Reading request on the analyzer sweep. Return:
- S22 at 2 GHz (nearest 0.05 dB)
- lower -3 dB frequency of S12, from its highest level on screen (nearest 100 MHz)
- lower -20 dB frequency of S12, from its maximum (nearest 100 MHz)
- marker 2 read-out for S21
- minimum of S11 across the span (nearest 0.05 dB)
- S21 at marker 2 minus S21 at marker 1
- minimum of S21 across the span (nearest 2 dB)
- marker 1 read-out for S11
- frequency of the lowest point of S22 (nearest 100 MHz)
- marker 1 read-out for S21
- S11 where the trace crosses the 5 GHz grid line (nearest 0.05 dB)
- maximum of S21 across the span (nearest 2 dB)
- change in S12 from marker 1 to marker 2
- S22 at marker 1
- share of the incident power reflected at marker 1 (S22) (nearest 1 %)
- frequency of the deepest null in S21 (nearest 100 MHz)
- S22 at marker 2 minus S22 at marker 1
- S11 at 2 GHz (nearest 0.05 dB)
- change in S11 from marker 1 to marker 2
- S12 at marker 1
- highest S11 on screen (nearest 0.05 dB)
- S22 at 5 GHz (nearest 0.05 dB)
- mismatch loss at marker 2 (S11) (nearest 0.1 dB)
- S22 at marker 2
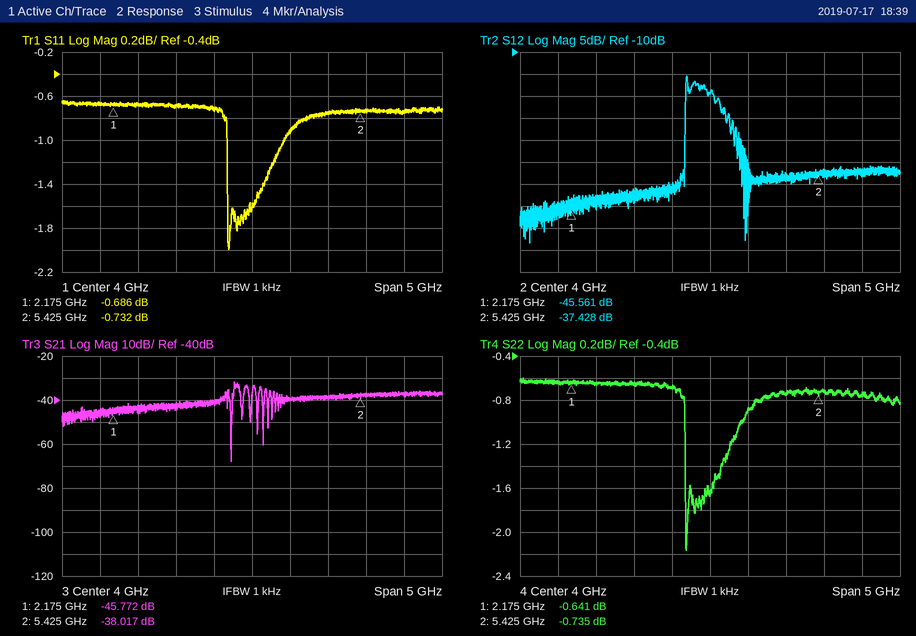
-0.65 dB
3.7 GHz
3.7 GHz
-38.017 dB
-2.00 dB
7.755 dB
-68 dB
-0.686 dB
3.7 GHz
-45.772 dB
-0.75 dB
-32 dB
8.133 dB
-0.641 dB
86 %
3.7 GHz
-0.094 dB
-0.65 dB
-0.046 dB
-45.561 dB
-0.65 dB
-0.75 dB
8.1 dB
-0.735 dB
